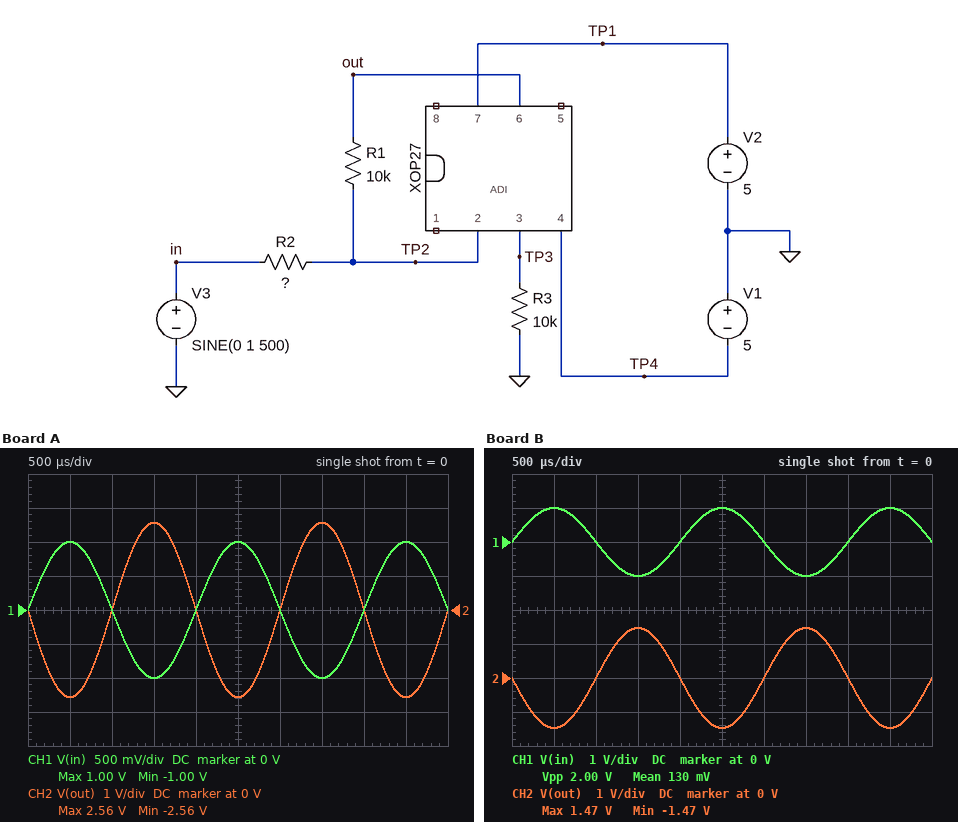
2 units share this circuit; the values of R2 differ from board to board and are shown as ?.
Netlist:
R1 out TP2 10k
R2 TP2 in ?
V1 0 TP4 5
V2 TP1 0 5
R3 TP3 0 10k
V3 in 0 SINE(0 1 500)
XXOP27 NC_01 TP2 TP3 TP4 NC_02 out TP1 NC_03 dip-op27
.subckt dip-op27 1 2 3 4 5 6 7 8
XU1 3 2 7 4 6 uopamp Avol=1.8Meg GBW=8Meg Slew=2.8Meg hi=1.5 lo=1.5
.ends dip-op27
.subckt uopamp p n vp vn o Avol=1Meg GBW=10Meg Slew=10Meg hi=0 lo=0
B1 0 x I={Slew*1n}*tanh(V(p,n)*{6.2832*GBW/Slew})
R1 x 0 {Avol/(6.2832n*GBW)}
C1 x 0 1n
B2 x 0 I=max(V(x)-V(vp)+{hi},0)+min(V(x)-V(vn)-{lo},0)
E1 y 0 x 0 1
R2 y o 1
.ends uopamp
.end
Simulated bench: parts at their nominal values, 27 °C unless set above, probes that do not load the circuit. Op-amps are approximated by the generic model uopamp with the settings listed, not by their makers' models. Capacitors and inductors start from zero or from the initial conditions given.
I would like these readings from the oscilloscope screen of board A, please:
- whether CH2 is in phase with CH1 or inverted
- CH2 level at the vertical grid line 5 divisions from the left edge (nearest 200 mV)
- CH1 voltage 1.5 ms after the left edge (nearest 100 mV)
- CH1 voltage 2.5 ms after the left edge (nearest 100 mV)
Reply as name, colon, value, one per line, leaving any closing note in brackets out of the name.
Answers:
whether CH2 is in phase with CH1 or inverted: inverted
CH2 level at the vertical grid line 5 divisions from the left edge: -2.6 V
CH1 voltage 1.5 ms after the left edge: -1.0 V
CH1 voltage 2.5 ms after the left edge: 1.0 V
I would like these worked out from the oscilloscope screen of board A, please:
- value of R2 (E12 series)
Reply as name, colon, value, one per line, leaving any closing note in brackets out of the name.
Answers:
value of R2: 3.9 kΩ
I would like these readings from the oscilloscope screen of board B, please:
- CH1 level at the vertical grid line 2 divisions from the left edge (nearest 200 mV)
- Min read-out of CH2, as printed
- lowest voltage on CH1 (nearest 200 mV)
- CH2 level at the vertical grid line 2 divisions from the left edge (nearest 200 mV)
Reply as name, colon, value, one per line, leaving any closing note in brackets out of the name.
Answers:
CH1 level at the vertical grid line 2 divisions from the left edge: 0 V
Min read-out of CH2, as printed: -1.47 V
lowest voltage on CH1: -1.0 V
CH2 level at the vertical grid line 2 divisions from the left edge: 0 V
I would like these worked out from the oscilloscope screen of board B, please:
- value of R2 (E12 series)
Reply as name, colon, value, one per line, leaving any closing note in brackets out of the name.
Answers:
value of R2: 6.8 kΩ
